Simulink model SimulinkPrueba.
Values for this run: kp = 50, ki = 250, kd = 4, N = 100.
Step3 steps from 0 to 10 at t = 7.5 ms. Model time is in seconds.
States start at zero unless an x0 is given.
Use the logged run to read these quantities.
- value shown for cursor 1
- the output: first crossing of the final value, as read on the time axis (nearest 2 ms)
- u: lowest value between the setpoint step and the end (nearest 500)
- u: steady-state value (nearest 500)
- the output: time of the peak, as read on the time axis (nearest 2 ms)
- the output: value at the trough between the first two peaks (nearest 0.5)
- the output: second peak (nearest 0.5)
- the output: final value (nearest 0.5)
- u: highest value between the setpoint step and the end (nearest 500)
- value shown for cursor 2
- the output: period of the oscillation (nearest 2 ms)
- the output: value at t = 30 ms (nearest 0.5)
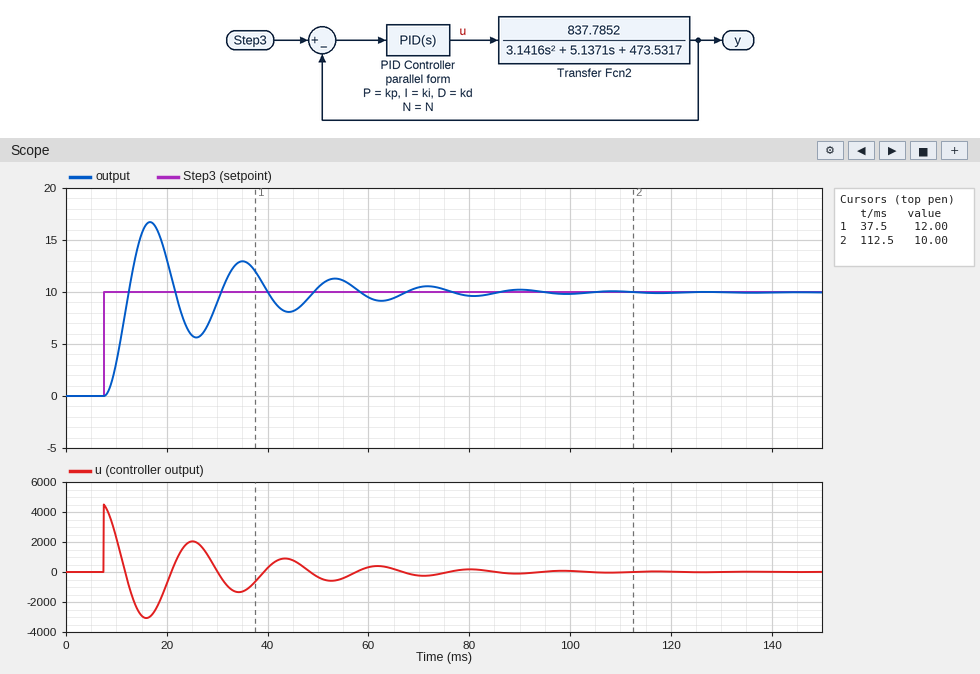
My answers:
12.00
12 ms
-3000
0
16 ms
5.5
13.0
10.0
4500
10.00
18 ms
9.0
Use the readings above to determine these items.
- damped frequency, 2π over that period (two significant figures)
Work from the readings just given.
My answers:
0.35 rad/ms
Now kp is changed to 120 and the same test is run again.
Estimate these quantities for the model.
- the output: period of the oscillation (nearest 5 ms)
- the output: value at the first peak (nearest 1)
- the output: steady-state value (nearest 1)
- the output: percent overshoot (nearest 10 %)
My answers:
15 ms
17
10
70 %
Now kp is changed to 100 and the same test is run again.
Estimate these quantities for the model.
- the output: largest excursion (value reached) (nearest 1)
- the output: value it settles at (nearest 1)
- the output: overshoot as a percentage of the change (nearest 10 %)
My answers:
17
10
70 %
